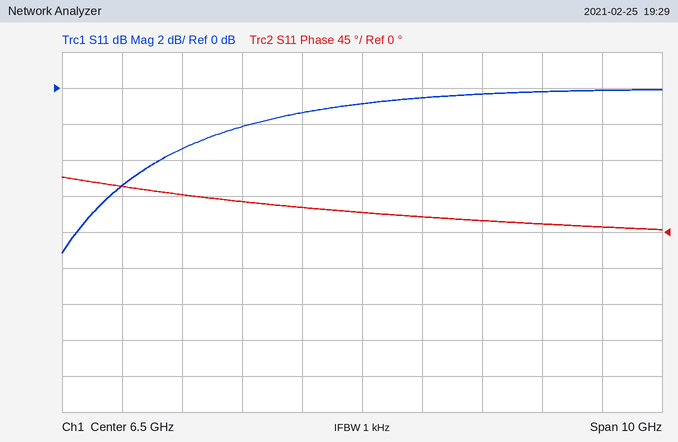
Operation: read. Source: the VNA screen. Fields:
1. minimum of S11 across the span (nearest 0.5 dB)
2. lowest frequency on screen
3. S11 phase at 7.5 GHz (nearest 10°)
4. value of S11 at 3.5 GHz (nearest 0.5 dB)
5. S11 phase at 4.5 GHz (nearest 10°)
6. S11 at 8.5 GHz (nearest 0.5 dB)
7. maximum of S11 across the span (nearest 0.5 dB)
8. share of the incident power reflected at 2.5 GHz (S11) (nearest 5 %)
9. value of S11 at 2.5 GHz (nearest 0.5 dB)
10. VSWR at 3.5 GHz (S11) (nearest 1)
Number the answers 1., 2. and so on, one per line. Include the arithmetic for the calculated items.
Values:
1. -9.0 dB
2. 1.5 GHz
3. 20°
4. -3.5 dB
5. 40°
6. -0.5 dB
7. 0.0 dB
8. 10^(-5.5/10) ≈ 28.2 %, so 30 % to the nearest 5 %
9. -5.5 dB
10. |Γ| = 10^(-3.5/20) = 0.6683; VSWR = (1 + 0.6683)/(1 − 0.6683) ≈ 5
